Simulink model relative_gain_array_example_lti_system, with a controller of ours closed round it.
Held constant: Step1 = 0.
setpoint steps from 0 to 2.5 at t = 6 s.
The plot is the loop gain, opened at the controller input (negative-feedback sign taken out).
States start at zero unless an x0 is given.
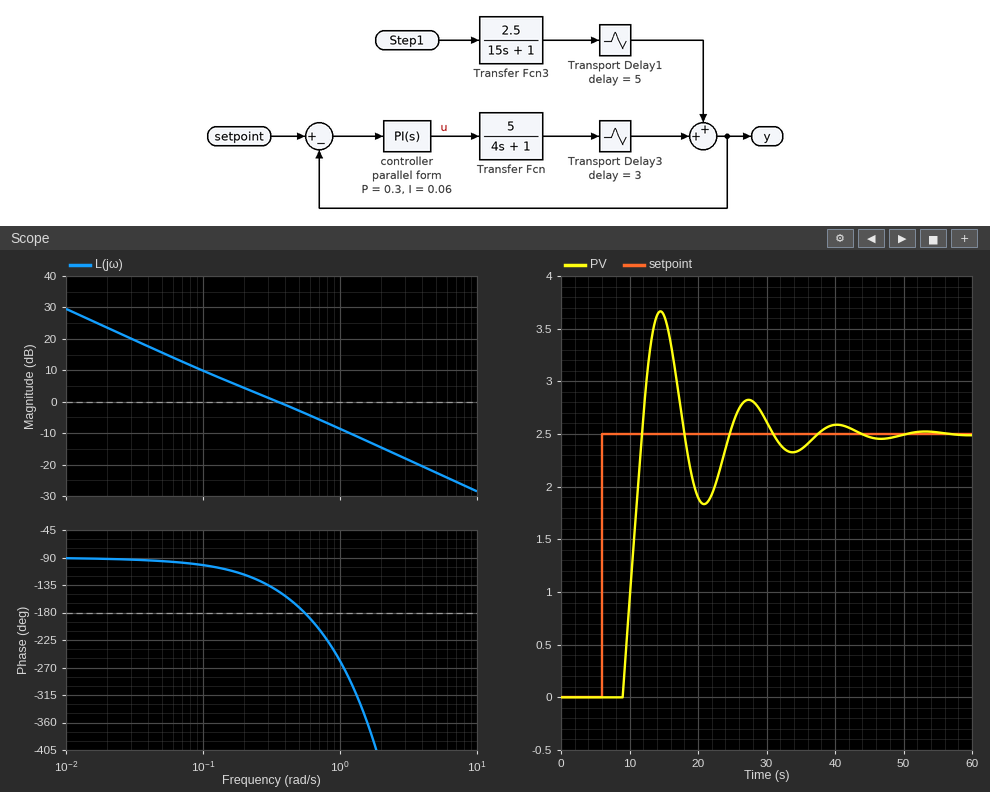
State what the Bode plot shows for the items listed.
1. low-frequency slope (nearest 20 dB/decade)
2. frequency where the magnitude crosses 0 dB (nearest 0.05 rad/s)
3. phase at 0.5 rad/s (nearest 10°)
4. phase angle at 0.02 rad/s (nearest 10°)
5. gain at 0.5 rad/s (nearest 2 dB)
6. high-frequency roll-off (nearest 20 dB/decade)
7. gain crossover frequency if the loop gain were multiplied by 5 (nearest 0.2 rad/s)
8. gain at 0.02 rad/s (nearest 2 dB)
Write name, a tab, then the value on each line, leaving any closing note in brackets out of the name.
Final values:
low-frequency slope	-20 dB/decade
frequency where the magnitude crosses 0 dB	0.35 rad/s
phase at 0.5 rad/s	-170°
phase angle at 0.02 rad/s	-90°
gain at 0.5 rad/s	-2 dB
high-frequency roll-off	-20 dB/decade
gain crossover frequency if the loop gain were multiplied by 5	1.8 rad/s
gain at 0.02 rad/s	24 dB
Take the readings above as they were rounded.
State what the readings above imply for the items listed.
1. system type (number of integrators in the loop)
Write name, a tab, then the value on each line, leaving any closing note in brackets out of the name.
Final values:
system type	1
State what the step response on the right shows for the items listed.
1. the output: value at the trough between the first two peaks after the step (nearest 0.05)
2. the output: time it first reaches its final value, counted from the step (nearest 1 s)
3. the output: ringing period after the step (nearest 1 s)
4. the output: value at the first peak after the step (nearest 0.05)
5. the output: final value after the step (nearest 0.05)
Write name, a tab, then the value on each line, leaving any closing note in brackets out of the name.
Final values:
the output: value at the trough between the first two peaks after the step	1.85
the output: time it first reaches its final value, counted from the step	6 s
the output: ringing period after the step	13 s
the output: value at the first peak after the step	3.65
the output: final value after the step	2.50
